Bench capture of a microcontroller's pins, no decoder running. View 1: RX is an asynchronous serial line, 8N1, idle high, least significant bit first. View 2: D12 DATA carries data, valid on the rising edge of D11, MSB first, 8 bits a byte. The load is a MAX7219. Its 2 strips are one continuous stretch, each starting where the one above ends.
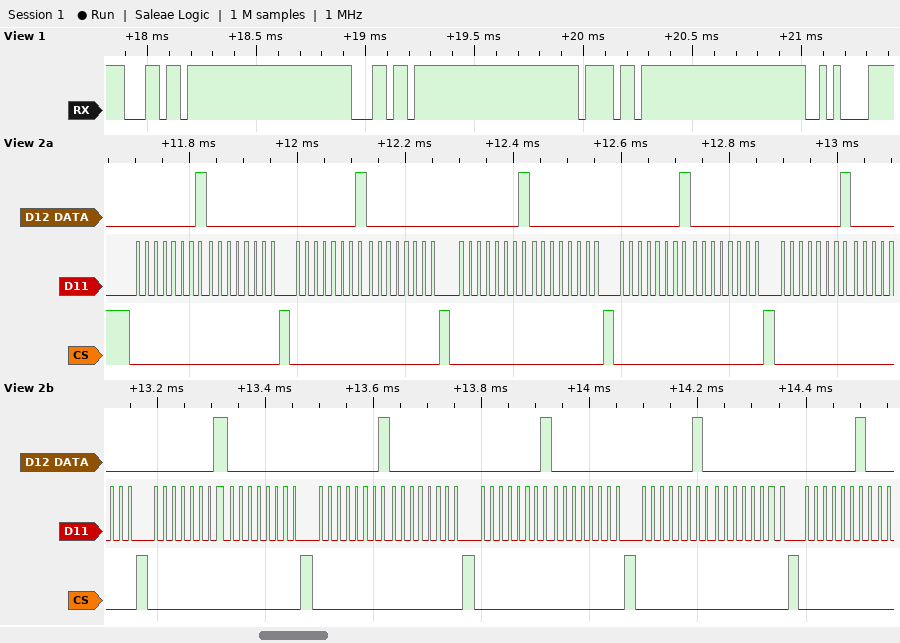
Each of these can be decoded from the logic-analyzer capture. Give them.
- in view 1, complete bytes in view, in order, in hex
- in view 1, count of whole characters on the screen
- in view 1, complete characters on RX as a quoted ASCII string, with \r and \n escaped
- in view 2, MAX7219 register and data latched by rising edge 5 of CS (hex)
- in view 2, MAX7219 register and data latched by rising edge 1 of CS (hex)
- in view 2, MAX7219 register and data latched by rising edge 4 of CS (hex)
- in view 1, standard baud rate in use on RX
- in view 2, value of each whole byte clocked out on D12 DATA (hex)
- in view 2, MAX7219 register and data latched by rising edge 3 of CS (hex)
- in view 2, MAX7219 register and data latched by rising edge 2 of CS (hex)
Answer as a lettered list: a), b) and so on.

a) 6C 6C 6F 0A
b) 4
c) "llo\n"
d) register 0x1, data 0x00
e) register 0x1, data 0x00
f) register 0x1, data 0x00
g) 31250 baud
h) 01 00 01 00 01 00 01 00 01 00 01 00 01 00 01 00 02 00 02
i) register 0x1, data 0x00
j) register 0x1, data 0x00
